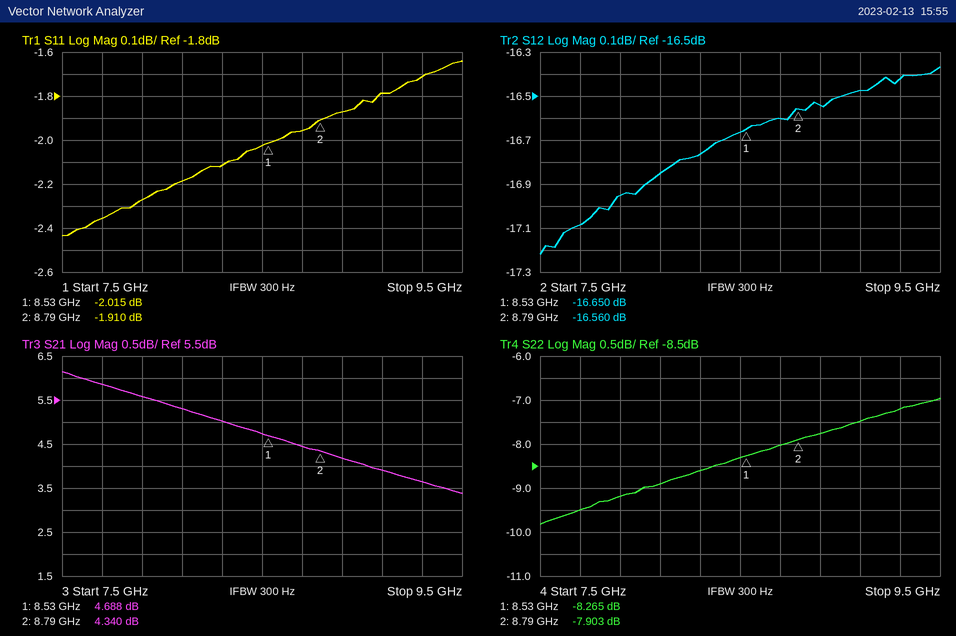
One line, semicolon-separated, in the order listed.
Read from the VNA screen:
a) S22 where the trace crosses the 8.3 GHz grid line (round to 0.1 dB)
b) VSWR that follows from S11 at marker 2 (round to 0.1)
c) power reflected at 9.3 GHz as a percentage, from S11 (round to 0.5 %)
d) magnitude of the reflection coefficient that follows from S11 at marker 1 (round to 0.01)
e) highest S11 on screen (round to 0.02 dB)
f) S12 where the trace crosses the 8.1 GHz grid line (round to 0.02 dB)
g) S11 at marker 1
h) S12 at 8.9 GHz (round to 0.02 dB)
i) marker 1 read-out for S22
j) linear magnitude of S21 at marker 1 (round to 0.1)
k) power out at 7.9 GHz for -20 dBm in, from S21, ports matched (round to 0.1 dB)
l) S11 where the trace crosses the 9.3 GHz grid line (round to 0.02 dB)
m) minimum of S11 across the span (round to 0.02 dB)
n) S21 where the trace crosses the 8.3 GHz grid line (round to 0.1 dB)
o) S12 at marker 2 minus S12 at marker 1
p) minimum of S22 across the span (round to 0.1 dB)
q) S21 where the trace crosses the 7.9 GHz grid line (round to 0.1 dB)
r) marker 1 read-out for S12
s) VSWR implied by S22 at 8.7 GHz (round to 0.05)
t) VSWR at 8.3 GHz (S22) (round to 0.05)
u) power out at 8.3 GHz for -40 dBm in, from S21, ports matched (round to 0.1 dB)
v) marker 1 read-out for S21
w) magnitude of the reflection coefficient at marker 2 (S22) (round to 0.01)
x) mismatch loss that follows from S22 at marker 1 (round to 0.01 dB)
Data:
-8.6 dB; 9.1; 67.5 %; 0.79; -1.64 dB; -16.86 dB; -2.015 dB; -16.54 dB; -8.265 dB; 1.7; -14.4 dBm; -1.72 dB; -2.44 dB; 5.0 dB; 0.090 dB; -9.8 dB; 5.6 dB; -16.650 dB; 2.30; 2.20; -35.0 dBm; 4.688 dB; 0.40; 0.70 dB
